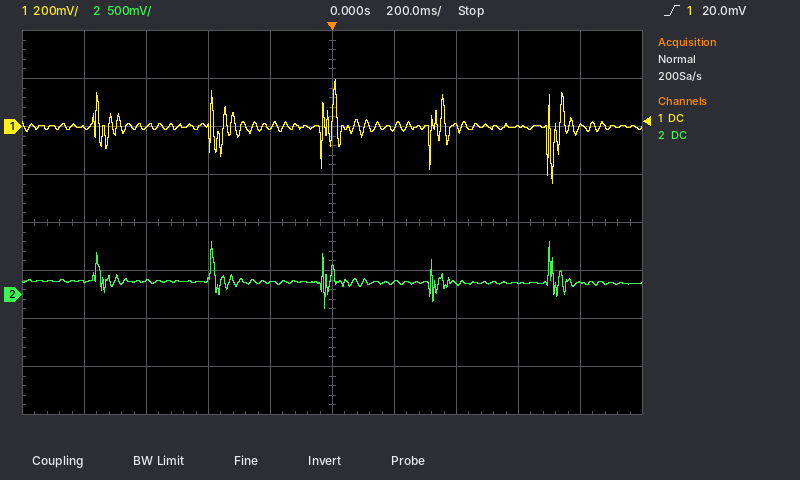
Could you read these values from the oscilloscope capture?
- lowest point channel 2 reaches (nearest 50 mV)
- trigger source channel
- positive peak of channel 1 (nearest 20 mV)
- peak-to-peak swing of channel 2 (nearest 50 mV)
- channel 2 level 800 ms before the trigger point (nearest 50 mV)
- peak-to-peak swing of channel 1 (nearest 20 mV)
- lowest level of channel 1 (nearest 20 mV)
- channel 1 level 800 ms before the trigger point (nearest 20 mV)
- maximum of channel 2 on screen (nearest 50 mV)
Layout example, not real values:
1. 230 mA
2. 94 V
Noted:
1. -150 mV
2. channel 1
3. 200 mV
4. 700 mV
5. 150 mV
6. 440 mV
7. -240 mV
8. 0 mV
9. 550 mV
